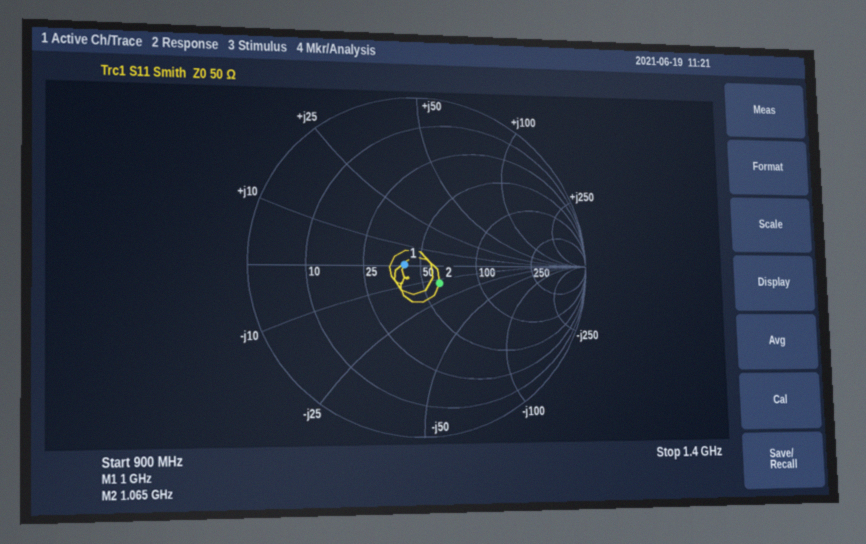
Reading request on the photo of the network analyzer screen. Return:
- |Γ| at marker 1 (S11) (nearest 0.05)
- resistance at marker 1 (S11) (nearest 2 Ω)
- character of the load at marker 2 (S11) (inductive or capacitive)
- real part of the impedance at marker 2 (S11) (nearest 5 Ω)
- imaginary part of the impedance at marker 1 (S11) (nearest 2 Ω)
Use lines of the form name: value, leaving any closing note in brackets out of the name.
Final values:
|Γ| at marker 1 (S11): 0.10
resistance at marker 1 (S11): 42 Ω
character of the load at marker 2 (S11): capacitive
real part of the impedance at marker 2 (S11): 60 Ω
imaginary part of the impedance at marker 1 (S11): 0 Ω
